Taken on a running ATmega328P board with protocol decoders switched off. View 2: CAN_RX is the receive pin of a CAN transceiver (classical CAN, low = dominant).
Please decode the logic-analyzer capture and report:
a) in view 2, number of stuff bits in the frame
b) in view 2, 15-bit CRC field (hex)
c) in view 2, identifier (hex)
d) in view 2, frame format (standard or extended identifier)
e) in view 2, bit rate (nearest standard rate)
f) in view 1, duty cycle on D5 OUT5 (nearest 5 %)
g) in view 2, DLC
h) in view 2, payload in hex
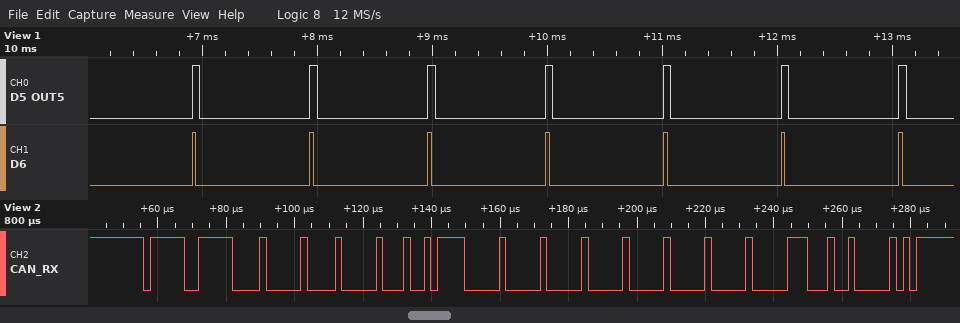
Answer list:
13
0x6240
0x7DF
standard
500 kbit/s
5 %
8
02 01 2F 00 00 00 00 00
